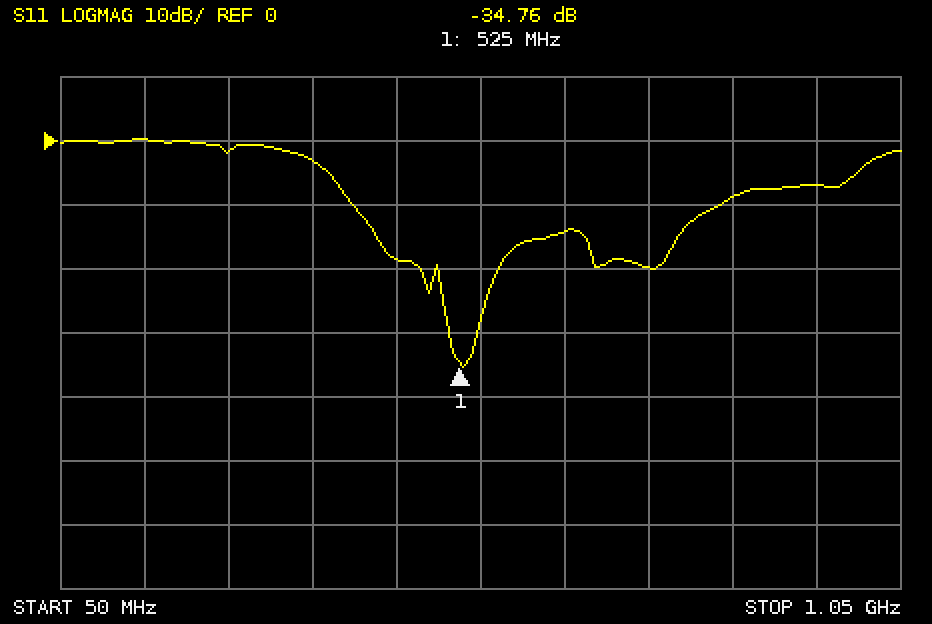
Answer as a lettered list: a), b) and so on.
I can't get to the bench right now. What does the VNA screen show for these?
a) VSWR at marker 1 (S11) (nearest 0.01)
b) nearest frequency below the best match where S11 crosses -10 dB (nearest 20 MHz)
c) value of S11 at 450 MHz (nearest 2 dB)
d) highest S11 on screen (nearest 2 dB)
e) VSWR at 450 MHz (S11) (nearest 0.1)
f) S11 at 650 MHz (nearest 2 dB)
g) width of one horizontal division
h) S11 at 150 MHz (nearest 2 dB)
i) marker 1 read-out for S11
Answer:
a) 1.04
b) 400 MHz
c) -18 dB
d) 0 dB
e) 1.3
f) -14 dB
g) 100 MHz
h) 0 dB
i) -34.76 dB
